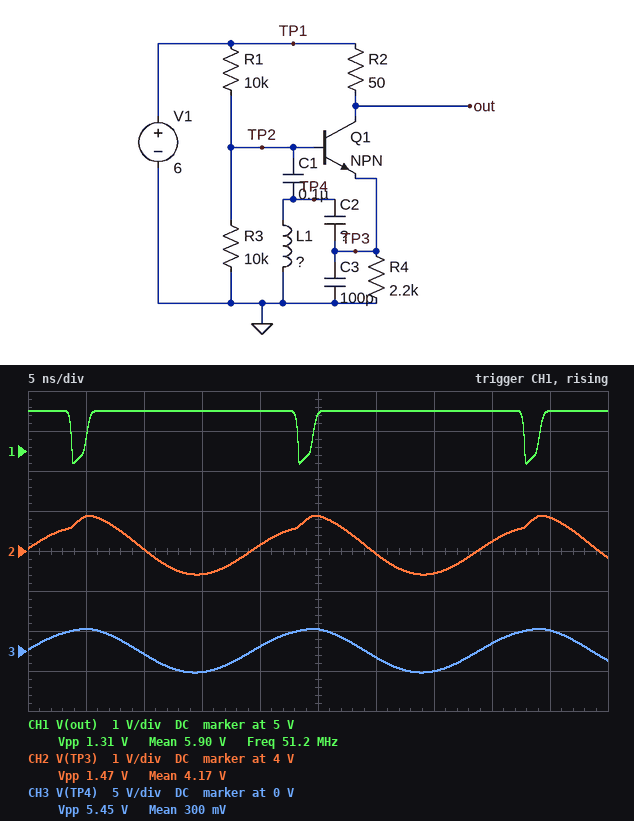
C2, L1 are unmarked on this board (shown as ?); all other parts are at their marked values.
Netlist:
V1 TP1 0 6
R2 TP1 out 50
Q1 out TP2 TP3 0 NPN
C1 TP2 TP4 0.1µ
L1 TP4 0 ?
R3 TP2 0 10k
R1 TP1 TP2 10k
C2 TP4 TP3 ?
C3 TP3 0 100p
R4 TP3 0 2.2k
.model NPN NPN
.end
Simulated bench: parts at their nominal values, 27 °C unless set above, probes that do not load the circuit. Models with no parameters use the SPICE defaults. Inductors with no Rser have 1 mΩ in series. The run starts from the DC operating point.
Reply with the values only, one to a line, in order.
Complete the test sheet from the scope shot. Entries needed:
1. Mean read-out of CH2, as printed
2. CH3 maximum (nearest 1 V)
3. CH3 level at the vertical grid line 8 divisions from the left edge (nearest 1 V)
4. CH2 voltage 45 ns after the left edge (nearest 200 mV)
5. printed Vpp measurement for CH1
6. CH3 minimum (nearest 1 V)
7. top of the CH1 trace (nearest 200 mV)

4.17 V
3 V
1 V
4.8 V
1.31 V
-3 V
6.0 V
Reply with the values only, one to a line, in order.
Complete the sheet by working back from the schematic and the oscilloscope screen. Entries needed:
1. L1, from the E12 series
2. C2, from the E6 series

390 nH
33 pF
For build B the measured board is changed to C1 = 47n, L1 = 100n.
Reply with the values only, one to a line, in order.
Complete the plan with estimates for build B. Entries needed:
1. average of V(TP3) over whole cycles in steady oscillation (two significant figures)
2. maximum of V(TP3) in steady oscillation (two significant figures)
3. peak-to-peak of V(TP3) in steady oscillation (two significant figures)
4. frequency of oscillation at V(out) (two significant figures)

4.0 V
4.7 V
1.3 V
100 MHz
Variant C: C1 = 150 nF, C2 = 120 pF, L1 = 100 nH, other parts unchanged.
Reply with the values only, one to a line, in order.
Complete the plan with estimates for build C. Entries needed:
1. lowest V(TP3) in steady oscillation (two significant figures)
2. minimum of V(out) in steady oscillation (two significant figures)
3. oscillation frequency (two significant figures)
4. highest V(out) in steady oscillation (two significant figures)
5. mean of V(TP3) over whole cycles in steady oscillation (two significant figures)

1.8 V
5.2 V
68 MHz
6.0 V
3.5 V
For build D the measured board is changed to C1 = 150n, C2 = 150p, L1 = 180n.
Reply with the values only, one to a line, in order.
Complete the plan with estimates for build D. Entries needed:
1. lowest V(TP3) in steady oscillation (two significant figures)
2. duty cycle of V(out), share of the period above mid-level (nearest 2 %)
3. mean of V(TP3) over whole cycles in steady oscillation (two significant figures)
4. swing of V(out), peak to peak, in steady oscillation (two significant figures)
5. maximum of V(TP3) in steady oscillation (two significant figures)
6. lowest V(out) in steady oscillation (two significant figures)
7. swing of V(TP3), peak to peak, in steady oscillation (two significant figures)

1.4 V
92 %
3.4 V
790 mV
5.3 V
5.2 V
3.9 V
